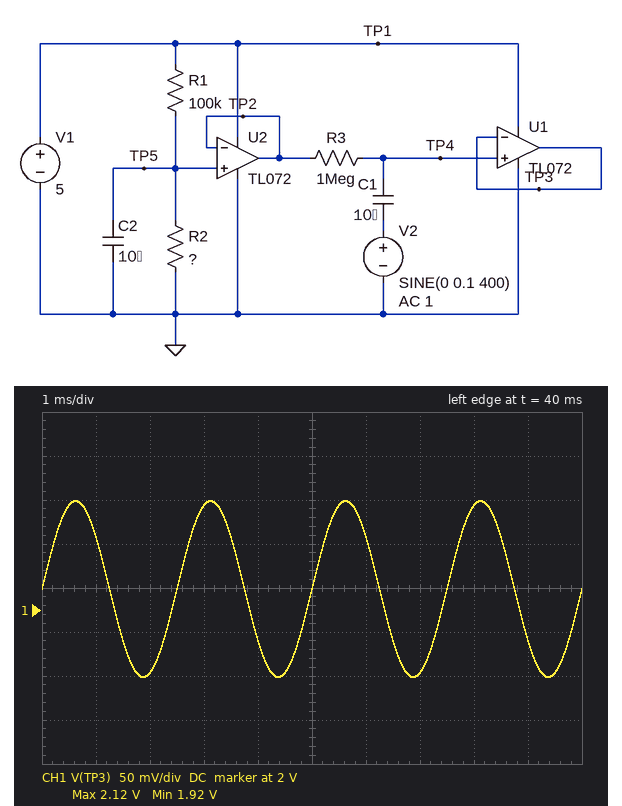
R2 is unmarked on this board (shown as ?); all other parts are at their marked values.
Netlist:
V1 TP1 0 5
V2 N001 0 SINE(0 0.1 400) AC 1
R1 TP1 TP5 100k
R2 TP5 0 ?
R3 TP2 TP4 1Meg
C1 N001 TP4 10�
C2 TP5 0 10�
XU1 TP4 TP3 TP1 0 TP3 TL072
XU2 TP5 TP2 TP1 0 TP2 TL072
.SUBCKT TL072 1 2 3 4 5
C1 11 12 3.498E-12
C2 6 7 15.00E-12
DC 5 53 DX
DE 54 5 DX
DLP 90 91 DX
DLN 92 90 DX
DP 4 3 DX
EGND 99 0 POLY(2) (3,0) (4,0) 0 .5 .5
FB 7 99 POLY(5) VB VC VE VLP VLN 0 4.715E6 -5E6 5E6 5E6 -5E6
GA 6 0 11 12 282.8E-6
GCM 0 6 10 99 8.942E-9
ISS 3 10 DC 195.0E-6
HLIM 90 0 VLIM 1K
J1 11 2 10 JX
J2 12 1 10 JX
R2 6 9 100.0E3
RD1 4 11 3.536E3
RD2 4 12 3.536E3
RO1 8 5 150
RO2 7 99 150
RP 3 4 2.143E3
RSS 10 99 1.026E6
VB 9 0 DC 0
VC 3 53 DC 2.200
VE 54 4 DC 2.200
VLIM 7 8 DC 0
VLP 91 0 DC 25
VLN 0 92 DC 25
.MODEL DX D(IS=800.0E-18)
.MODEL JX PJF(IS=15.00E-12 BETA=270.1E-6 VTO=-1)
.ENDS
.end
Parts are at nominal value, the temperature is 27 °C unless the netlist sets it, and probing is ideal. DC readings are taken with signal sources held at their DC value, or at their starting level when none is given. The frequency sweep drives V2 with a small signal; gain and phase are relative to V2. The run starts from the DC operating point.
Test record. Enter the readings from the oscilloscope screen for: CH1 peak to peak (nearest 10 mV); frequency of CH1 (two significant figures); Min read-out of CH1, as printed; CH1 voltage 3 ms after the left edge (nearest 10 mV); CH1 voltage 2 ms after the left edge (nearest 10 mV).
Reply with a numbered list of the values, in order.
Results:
1. 200 mV
2. 400 Hz
3. 1.92 V
4. 2.12 V
5. 1.93 V
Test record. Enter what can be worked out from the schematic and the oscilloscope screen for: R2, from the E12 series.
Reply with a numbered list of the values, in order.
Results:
1. 68 kΩ
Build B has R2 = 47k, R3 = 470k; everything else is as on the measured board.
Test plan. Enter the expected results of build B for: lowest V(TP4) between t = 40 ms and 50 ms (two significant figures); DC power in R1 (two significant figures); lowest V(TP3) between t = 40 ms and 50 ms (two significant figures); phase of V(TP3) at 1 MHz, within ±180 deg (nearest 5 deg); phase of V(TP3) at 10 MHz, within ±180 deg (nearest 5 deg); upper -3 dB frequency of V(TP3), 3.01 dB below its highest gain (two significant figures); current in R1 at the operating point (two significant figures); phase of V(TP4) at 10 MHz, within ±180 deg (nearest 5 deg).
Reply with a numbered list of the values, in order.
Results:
1. 1.5 V
2. 120 µW
3. 1.6 V
4. -80 deg
5. -145 deg
6. 340 kHz
7. 34 µA
8. 0 deg
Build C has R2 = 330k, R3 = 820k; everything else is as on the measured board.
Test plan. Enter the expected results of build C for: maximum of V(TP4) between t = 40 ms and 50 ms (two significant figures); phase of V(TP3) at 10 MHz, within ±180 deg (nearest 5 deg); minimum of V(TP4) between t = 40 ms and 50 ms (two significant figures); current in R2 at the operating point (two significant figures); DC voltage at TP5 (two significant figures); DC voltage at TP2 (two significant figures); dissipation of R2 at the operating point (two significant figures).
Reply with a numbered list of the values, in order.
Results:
1. 3.6 V
2. -145 deg
3. 3.4 V
4. 12 µA
5. 3.8 V
6. 3.5 V
7. 45 µW
